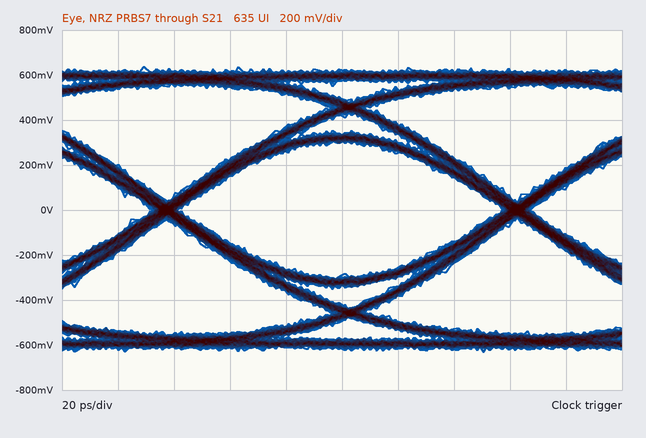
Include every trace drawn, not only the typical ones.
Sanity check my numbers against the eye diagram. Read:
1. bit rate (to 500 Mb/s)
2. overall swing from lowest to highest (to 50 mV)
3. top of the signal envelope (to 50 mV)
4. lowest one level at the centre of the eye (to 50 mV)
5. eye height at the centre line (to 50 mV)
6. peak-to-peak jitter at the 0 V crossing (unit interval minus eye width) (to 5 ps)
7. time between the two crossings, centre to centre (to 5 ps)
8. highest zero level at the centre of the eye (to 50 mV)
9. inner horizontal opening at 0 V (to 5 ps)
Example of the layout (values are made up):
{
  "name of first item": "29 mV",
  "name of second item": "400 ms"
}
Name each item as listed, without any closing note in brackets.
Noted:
{
  "bit rate": "8.0 Gb/s",
  "overall swing from lowest to highest": "1.25 V",
  "top of the signal envelope": "650 mV",
  "lowest one level at the centre of the eye": "300 mV",
  "eye height at the centre line": "600 mV",
  "peak-to-peak jitter at the 0 V crossing (unit interval minus eye width)": "10 ps",
  "time between the two crossings, centre to centre": "125 ps",
  "highest zero level at the centre of the eye": "-300 mV",
  "inner horizontal opening at 0 V": "115 ps"
}
